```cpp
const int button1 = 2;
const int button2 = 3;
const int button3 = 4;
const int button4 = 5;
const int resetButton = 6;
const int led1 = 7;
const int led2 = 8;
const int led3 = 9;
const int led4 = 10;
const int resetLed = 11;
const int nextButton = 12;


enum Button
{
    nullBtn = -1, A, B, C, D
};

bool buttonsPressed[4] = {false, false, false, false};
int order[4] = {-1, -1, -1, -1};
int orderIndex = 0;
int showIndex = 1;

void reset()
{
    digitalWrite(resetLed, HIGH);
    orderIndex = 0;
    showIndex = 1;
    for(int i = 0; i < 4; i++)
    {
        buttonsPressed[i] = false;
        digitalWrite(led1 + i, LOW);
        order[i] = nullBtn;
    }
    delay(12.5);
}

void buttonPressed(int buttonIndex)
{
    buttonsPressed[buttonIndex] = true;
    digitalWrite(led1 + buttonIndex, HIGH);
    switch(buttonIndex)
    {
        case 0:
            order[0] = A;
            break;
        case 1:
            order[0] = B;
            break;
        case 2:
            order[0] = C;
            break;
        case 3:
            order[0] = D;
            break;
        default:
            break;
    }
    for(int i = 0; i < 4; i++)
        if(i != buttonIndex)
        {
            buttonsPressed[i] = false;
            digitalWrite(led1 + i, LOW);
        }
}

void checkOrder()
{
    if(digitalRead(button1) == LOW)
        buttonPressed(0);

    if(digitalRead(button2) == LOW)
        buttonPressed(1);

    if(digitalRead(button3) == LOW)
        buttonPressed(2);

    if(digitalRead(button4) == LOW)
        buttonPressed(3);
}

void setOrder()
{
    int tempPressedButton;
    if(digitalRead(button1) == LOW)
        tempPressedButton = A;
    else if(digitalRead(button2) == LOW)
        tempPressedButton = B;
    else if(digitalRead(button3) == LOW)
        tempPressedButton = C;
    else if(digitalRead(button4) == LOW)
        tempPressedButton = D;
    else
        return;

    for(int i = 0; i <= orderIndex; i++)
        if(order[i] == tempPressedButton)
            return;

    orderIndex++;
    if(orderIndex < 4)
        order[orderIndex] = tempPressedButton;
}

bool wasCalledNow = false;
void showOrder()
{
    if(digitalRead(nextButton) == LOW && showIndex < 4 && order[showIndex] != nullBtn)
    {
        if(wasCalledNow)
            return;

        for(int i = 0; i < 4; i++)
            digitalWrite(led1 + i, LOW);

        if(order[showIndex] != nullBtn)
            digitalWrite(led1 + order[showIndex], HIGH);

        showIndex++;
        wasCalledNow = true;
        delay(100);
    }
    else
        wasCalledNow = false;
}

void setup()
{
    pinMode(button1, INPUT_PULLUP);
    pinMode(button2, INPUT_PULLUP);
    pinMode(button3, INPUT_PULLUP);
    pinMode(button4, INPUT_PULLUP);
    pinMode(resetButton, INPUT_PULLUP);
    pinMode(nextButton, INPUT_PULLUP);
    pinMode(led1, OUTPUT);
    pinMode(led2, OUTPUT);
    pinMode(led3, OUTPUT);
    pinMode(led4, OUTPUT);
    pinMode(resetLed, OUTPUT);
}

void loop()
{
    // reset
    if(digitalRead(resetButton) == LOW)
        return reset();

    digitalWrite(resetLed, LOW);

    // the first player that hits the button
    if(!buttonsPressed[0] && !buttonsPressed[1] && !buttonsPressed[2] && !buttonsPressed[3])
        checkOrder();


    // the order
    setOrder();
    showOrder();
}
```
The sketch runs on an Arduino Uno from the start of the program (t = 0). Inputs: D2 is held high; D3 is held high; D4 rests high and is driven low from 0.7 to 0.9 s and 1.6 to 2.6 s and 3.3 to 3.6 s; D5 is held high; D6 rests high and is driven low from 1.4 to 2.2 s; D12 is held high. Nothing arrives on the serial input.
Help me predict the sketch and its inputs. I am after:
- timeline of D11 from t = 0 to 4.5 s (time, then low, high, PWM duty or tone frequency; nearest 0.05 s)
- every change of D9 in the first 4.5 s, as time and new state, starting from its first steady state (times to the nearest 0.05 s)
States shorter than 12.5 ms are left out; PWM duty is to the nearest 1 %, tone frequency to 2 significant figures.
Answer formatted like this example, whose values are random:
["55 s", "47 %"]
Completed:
["0 s low; 1.4 s high; 2.2 s low", "0 s low; 0.7 s high; 1.4 s low; 2.2 s high"]
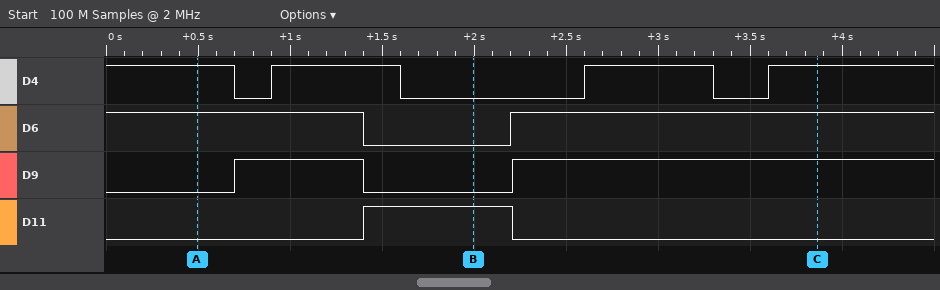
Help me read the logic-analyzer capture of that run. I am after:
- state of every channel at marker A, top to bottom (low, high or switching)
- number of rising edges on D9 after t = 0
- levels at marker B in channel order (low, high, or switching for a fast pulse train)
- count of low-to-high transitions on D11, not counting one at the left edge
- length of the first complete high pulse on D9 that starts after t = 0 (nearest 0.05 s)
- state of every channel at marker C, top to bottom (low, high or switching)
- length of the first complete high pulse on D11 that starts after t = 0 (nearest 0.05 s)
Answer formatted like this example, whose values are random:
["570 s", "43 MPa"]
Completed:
["D4 high, D6 high, D9 low, D11 low", "2", "D4 low, D6 low, D9 low, D11 high", "1", "0.70 s", "D4 high, D6 high, D9 high, D11 low", "0.80 s"]
